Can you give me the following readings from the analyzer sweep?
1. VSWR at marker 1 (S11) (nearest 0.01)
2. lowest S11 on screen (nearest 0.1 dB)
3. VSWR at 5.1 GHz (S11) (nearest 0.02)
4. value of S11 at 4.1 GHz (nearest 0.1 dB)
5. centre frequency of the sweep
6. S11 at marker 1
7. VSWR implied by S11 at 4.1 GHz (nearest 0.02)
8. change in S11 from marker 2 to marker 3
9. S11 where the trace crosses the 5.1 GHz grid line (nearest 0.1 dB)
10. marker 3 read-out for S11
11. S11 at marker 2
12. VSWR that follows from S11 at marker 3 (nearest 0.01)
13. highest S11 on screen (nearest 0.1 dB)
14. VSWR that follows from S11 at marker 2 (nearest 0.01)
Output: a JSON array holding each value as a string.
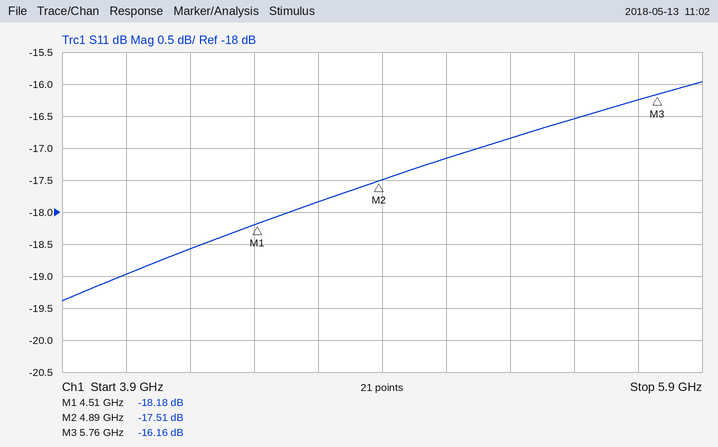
["1.28", "-19.4 dB", "1.32", "-19.0 dB", "4.9 GHz", "-18.18 dB", "1.26", "1.35 dB", "-17.2 dB", "-16.16 dB", "-17.51 dB", "1.37", "-16.0 dB", "1.31"]
